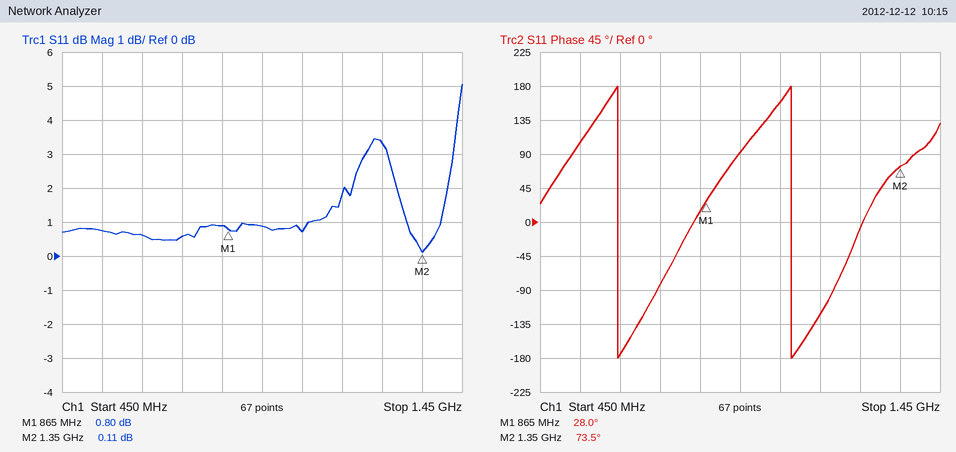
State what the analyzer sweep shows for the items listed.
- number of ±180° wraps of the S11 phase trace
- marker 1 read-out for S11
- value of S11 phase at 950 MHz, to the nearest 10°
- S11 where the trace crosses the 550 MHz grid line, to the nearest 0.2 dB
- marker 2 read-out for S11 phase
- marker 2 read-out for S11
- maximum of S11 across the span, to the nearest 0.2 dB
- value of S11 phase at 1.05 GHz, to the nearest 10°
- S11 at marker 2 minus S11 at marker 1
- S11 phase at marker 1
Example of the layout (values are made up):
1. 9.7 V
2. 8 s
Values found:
1. 2
2. 0.80 dB
3. 90°
4. 0.8 dB
5. 73.5°
6. 0.11 dB
7. 5.0 dB
8. 160°
9. -0.69 dB
10. 28.0°
